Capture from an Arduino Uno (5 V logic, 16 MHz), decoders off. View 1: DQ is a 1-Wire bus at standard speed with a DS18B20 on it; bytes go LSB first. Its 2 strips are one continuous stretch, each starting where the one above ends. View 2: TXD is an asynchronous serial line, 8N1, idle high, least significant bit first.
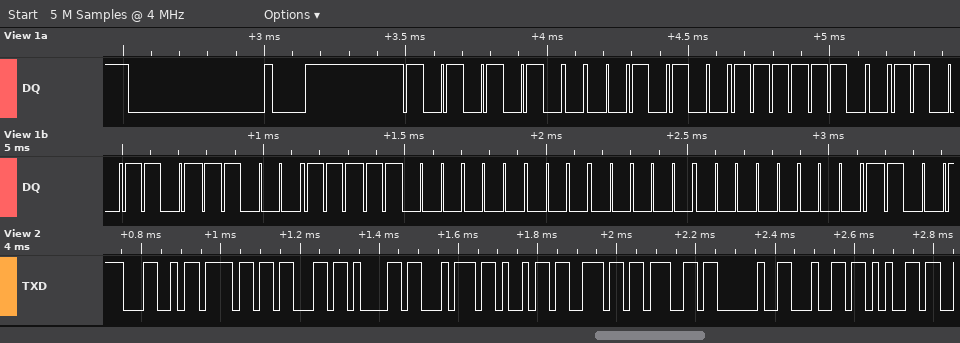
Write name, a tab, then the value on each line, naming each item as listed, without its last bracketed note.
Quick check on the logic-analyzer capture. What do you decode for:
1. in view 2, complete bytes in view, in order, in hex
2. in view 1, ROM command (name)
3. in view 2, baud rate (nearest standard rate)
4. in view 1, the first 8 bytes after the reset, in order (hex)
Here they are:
in view 2, complete bytes in view, in order, in hex	4C 6F 63 61 74 69 6E 67 20 64 65
in view 1, ROM command	Match ROM
in view 2, baud rate	57600 baud
in view 1, the first 8 bytes after the reset, in order	55 28 3F B3 E3 03 00 00
